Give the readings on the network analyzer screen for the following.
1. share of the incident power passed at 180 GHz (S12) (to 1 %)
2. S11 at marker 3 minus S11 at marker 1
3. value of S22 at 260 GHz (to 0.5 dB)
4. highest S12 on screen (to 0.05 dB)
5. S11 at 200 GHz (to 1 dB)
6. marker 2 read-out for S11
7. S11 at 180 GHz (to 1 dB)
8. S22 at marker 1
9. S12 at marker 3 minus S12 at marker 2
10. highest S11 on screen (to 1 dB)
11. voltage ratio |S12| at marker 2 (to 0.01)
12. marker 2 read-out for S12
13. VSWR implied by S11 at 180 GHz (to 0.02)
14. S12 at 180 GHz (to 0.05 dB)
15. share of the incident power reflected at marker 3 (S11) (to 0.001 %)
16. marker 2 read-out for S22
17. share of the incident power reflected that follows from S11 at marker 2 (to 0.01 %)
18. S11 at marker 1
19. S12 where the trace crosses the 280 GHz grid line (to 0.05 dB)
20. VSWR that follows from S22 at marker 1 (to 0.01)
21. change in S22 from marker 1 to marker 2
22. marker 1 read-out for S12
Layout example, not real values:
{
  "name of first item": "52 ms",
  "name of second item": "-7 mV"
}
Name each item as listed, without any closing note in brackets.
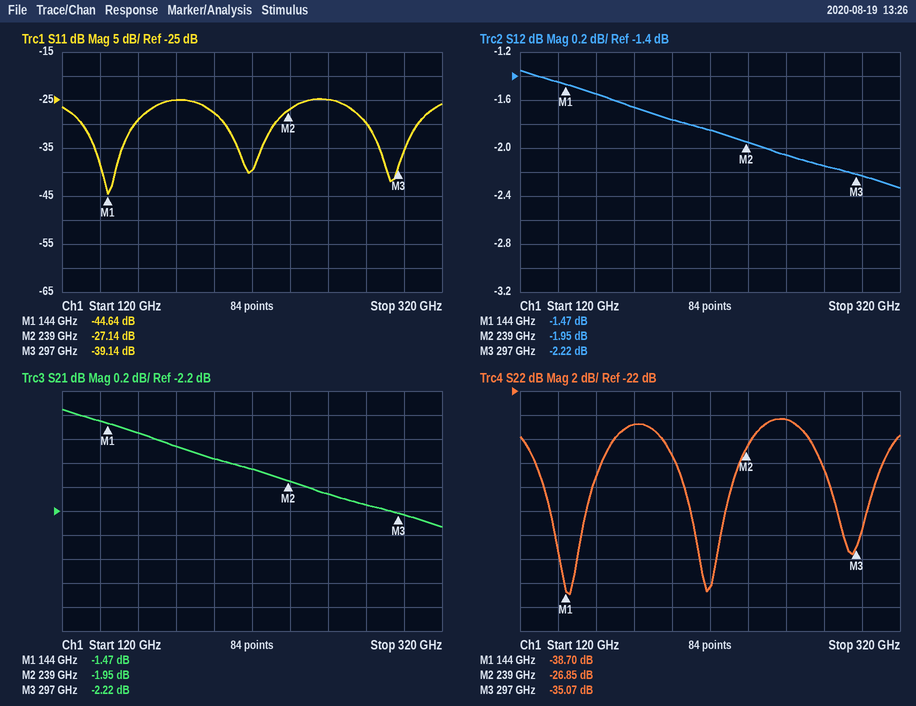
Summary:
{
  "share of the incident power passed at 180 GHz (S12)": "68 %",
  "S11 at marker 3 minus S11 at marker 1": "5.50 dB",
  "value of S22 at 260 GHz": "-24.5 dB",
  "highest S12 on screen": "-1.35 dB",
  "S11 at 200 GHz": "-28 dB",
  "marker 2 read-out for S11": "-27.14 dB",
  "S11 at 180 GHz": "-25 dB",
  "S22 at marker 1": "-38.70 dB",
  "S12 at marker 3 minus S12 at marker 2": "-0.27 dB",
  "highest S11 on screen": "-25 dB",
  "voltage ratio |S12| at marker 2": "0.80",
  "marker 2 read-out for S12": "-1.95 dB",
  "VSWR implied by S11 at 180 GHz": "1.12",
  "S12 at 180 GHz": "-1.65 dB",
  "share of the incident power reflected at marker 3 (S11)": "0.012 %",
  "marker 2 read-out for S22": "-26.85 dB",
  "share of the incident power reflected that follows from S11 at marker 2": "0.19 %",
  "S11 at marker 1": "-44.64 dB",
  "S12 where the trace crosses the 280 GHz grid line": "-2.15 dB",
  "VSWR that follows from S22 at marker 1": "1.02",
  "change in S22 from marker 1 to marker 2": "11.85 dB",
  "marker 1 read-out for S12": "-1.47 dB"
}
